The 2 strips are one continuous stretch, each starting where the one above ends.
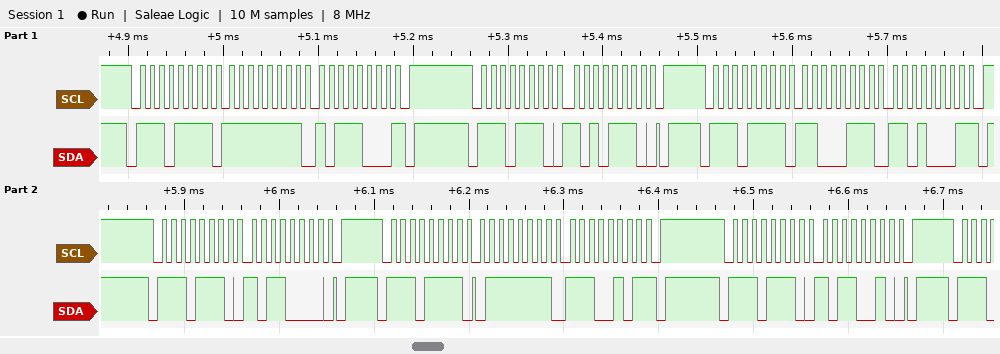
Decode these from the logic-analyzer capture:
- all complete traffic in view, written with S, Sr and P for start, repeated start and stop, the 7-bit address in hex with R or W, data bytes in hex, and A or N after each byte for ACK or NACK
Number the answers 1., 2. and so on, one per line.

1. S 77R A FF A B8 N P S 77W A AE A P S 77R A C7 A D1 N P S 77W A B0 A P S 77R A 7F A E5 N P S 77W A B2 A P
